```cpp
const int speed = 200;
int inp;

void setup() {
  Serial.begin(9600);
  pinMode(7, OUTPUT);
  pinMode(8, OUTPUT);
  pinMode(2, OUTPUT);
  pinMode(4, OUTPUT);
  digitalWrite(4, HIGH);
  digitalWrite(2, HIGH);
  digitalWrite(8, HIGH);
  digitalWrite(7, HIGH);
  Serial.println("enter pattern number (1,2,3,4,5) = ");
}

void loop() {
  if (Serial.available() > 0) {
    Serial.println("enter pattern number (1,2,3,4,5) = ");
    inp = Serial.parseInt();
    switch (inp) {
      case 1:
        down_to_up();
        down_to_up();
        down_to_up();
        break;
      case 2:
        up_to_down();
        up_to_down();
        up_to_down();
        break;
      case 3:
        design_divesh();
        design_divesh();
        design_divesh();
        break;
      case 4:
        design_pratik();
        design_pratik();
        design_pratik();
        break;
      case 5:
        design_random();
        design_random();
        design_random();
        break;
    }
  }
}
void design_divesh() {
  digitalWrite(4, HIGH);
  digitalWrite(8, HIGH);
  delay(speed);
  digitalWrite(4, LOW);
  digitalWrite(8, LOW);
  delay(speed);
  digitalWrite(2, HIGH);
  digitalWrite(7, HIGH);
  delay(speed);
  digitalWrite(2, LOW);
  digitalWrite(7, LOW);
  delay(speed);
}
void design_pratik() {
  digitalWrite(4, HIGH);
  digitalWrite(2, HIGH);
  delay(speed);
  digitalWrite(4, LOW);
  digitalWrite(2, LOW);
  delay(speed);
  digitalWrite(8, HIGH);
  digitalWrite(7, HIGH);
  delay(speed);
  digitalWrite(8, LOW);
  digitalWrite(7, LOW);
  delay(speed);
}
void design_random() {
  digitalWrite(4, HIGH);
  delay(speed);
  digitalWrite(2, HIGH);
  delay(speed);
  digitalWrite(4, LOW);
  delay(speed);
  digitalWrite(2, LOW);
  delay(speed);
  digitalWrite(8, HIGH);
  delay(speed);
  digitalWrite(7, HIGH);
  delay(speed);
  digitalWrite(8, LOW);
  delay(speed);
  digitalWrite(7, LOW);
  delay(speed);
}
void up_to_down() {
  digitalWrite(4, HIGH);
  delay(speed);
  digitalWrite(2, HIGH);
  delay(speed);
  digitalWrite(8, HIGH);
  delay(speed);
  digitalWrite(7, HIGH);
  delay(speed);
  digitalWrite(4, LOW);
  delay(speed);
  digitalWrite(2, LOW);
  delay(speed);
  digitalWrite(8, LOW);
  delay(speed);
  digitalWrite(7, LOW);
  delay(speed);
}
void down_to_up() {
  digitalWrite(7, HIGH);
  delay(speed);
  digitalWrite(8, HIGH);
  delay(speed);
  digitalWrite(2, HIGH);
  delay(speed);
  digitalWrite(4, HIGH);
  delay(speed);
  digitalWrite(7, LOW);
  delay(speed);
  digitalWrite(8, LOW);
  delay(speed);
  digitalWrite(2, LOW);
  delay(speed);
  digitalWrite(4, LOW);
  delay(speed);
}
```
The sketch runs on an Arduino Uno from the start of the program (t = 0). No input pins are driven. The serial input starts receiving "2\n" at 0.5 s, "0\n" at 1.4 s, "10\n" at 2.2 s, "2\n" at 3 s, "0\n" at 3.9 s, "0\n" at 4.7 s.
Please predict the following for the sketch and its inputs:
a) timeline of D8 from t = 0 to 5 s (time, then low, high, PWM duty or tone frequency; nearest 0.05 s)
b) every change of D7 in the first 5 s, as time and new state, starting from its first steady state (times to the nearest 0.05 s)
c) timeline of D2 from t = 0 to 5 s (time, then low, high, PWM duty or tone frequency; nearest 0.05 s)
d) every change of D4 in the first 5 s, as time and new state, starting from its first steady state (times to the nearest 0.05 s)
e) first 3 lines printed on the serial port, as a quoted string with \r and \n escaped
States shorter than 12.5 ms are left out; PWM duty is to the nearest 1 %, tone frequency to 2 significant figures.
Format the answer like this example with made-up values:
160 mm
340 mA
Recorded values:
0 s high; 1.7 s low; 2.5 s high; 3.3 s low; 4.1 s high; 4.9 s low
0 s high; 1.9 s low; 2.7 s high; 3.5 s low; 4.3 s high
0 s high; 1.5 s low; 2.3 s high; 3.1 s low; 3.9 s high; 4.7 s low
0 s high; 1.3 s low; 2.1 s high; 2.9 s low; 3.7 s high; 4.5 s low
"enter pattern number (1,2,3,4,5) = \r\nenter pattern number (1,2,3,4,5) = \r\nenter pattern number (1,2,3,4,5) = \r\n"
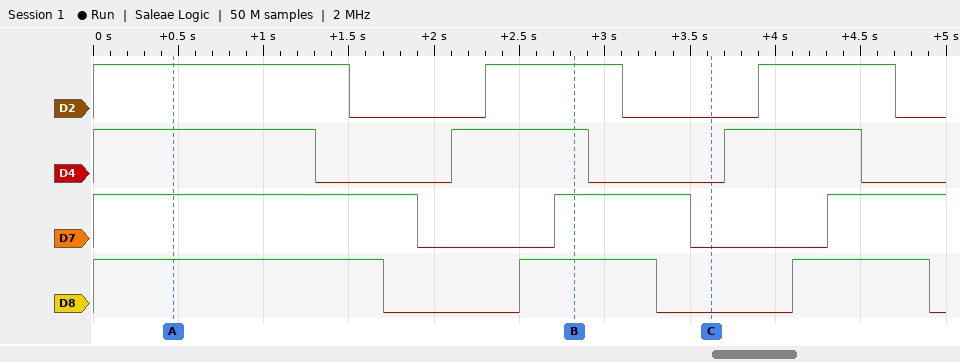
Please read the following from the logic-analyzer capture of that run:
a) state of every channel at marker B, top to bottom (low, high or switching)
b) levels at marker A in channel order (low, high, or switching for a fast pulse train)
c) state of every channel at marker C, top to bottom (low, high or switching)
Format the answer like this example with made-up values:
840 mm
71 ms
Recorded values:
D2 high, D4 high, D7 high, D8 high
D2 high, D4 high, D7 high, D8 high
D2 low, D4 low, D7 low, D8 low
